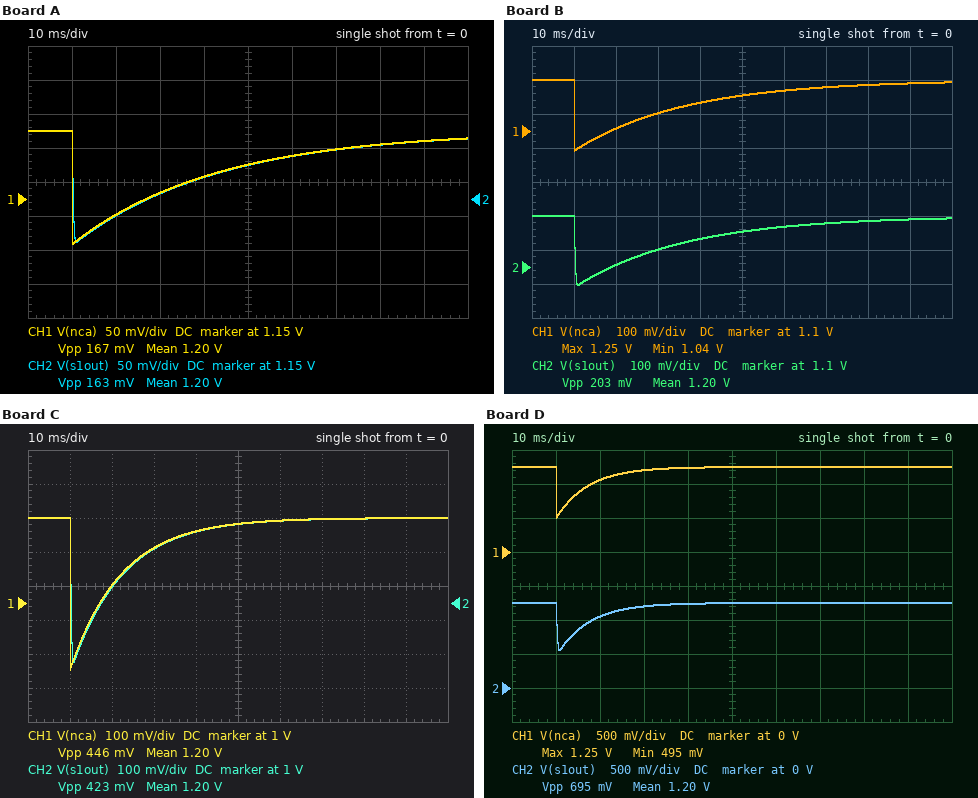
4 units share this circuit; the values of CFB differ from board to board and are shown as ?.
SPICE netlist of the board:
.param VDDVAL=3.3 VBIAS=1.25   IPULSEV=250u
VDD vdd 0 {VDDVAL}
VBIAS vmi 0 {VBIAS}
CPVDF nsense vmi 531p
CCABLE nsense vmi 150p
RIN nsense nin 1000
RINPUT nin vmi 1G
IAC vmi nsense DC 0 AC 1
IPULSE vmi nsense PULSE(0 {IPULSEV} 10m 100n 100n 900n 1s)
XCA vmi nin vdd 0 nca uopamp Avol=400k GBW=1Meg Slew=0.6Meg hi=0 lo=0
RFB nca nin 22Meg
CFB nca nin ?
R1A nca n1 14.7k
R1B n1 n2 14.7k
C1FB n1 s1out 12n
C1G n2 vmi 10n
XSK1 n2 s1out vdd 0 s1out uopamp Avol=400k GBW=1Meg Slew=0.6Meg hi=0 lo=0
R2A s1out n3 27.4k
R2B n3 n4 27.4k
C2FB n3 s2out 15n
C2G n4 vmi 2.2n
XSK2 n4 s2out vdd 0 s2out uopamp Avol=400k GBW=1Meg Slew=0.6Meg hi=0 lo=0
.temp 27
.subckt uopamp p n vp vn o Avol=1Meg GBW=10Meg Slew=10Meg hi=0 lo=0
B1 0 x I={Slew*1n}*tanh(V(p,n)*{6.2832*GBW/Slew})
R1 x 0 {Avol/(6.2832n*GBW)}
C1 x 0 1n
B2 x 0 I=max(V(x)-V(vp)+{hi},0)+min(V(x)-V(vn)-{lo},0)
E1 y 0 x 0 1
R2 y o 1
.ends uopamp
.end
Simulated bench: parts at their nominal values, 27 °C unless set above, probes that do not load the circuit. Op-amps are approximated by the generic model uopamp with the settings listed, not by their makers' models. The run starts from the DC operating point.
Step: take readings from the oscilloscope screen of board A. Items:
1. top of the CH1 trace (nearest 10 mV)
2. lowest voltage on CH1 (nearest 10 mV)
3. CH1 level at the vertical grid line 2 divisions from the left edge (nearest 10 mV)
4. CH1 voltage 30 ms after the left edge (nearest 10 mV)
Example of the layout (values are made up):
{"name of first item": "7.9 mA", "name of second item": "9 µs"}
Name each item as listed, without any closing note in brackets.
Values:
{"top of the CH1 trace": "1.25 V", "lowest voltage on CH1": "1.08 V", "CH1 level at the vertical grid line 2 divisions from the left edge": "1.13 V", "CH1 voltage 30 ms after the left edge": "1.16 V"}
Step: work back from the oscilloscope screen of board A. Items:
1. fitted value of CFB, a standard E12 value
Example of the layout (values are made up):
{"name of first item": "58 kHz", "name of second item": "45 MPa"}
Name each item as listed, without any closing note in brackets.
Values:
{"fitted value of CFB, a standard E12 value": "1.5 nF"}
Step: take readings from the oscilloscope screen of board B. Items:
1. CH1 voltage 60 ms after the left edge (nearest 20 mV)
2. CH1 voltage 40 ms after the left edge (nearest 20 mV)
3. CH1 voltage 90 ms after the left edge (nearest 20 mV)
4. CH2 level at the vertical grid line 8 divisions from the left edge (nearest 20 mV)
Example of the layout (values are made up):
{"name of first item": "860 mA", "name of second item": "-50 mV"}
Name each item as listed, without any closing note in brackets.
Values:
{"CH1 voltage 60 ms after the left edge": "1.22 V", "CH1 voltage 40 ms after the left edge": "1.18 V", "CH1 voltage 90 ms after the left edge": "1.24 V", "CH2 level at the vertical grid line 8 divisions from the left edge": "1.24 V"}
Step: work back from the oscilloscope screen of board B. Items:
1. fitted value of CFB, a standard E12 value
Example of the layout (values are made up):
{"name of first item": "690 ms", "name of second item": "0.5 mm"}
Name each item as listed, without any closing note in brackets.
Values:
{"fitted value of CFB, a standard E12 value": "1.2 nF"}
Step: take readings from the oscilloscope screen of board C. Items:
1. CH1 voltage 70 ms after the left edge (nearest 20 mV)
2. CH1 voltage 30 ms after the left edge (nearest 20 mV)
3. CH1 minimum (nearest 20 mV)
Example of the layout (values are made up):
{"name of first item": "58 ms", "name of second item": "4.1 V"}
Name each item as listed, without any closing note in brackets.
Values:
{"CH1 voltage 70 ms after the left edge": "1.24 V", "CH1 voltage 30 ms after the left edge": "1.16 V", "CH1 minimum": "800 mV"}
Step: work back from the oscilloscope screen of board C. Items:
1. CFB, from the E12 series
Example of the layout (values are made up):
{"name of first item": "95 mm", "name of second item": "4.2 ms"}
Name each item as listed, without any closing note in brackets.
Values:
{"CFB, from the E12 series": "560 pF"}
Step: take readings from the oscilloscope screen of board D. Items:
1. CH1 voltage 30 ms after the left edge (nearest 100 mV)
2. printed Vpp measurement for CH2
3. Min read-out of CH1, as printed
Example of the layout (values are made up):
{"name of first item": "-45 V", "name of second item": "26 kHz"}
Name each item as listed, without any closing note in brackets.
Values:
{"CH1 voltage 30 ms after the left edge": "1.2 V", "printed Vpp measurement for CH2": "695 mV", "Min read-out of CH1, as printed": "495 mV"}
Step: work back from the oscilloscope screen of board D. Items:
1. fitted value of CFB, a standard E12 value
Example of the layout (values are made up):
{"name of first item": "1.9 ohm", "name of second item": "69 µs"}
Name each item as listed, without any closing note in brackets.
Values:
{"fitted value of CFB, a standard E12 value": "330 pF"}
